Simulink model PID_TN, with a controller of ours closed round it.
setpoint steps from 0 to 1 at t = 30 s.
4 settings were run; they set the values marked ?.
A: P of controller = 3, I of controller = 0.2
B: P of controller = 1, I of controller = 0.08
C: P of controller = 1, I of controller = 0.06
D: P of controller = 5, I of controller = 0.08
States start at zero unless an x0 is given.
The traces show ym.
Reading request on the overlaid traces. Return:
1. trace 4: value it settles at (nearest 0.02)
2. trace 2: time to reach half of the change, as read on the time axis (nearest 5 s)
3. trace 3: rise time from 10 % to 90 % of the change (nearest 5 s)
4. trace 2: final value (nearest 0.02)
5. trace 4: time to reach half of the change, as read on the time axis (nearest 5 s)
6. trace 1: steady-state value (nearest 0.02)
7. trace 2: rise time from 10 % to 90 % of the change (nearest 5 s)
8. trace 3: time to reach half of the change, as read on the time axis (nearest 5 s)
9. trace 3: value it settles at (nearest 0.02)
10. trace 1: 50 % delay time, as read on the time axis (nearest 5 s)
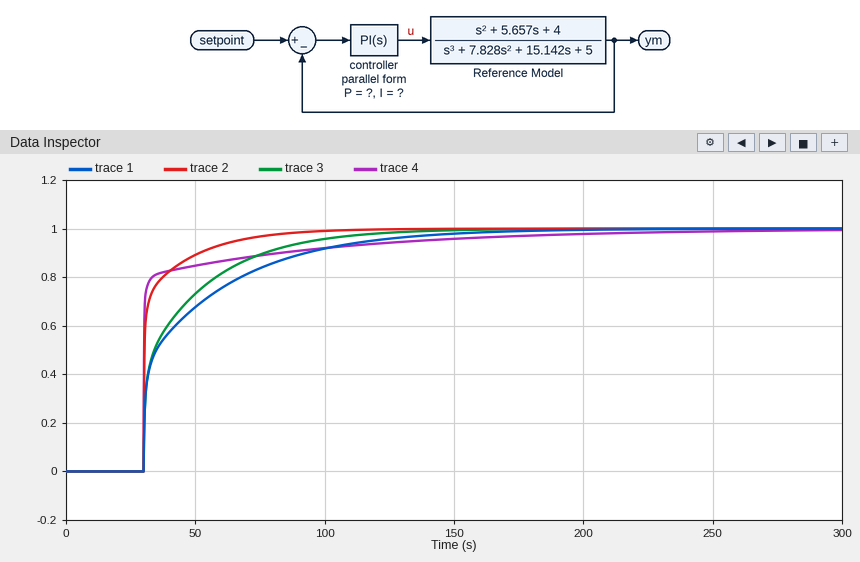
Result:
1.00
30 s
45 s
1.00
30 s
1.00
20 s
35 s
1.00
35 s
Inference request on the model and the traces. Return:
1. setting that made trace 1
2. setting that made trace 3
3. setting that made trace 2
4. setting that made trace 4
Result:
C
B
A
D
